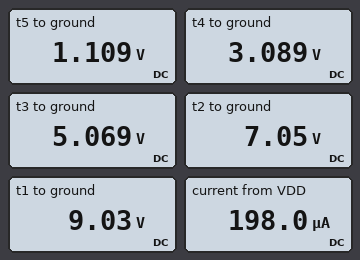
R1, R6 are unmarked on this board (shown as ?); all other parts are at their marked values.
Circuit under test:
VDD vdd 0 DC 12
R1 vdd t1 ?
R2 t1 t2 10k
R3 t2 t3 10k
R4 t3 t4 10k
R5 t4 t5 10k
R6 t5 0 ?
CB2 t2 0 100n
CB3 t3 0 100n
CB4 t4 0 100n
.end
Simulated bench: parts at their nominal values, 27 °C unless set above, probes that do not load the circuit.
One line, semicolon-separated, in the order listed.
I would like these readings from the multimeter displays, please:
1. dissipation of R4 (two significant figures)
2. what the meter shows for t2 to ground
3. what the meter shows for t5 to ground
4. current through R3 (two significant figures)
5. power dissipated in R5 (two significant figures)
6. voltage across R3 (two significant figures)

390 µW; 7.05 V; 1.109 V; 200 µA; 390 µW; 2.0 V
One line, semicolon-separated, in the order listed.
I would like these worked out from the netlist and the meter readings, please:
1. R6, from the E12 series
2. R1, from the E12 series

5.6 kΩ; 15 kΩ
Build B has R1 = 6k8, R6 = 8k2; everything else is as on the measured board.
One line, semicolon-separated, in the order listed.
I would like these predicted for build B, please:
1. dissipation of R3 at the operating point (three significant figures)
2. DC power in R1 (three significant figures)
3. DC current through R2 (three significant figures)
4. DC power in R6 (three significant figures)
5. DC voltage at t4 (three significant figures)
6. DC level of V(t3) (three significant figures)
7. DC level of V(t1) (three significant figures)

476 µW; 324 µW; 218 µA; 390 µW; 3.97 V; 6.15 V; 10.5 V
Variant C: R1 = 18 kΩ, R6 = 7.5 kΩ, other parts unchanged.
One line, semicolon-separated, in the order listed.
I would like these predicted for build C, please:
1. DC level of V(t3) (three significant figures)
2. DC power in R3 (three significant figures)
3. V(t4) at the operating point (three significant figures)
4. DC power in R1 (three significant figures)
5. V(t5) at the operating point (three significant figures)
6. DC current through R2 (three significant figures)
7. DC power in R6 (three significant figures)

5.04 V; 336 µW; 3.21 V; 604 µW; 1.37 V; 183 µA; 252 µW
